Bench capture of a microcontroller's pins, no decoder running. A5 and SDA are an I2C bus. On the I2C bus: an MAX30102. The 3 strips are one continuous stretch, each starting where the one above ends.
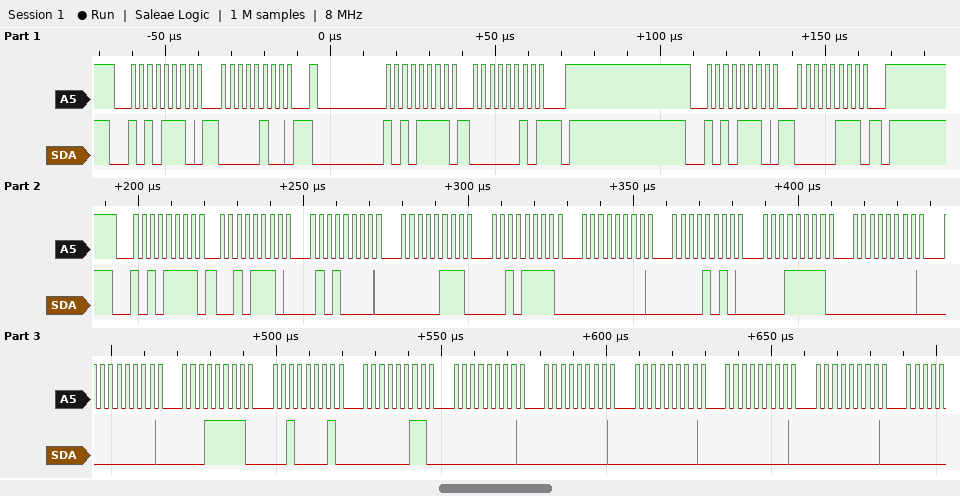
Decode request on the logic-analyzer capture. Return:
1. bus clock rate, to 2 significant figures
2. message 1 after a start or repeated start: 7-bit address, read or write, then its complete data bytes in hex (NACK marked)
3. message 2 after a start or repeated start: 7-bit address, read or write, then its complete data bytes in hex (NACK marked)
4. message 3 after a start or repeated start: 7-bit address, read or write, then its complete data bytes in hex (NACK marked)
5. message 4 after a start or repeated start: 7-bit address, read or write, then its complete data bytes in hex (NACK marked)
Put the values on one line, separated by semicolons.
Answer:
400 kHz; 0x57 write: 04; 0x57 read: 02 NACK; 0x57 write: 07; 0x57 read: 2E 50 07 2F 00 0A 1F 00 00 1F 21 03 00 00 00 00 00
